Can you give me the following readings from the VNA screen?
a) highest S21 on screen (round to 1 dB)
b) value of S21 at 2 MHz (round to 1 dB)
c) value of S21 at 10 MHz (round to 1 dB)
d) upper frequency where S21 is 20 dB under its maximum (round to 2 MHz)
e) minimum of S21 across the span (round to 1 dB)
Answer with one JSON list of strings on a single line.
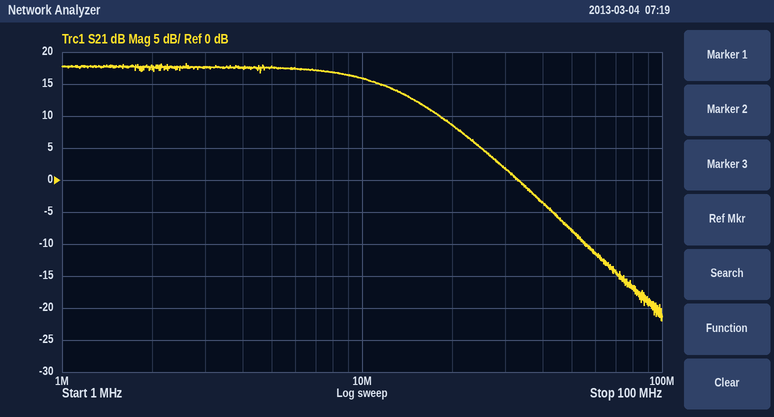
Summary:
["18 dB", "18 dB", "16 dB", "36 MHz", "-22 dB"]
